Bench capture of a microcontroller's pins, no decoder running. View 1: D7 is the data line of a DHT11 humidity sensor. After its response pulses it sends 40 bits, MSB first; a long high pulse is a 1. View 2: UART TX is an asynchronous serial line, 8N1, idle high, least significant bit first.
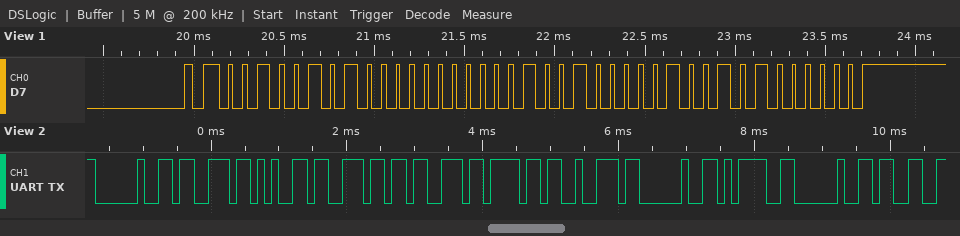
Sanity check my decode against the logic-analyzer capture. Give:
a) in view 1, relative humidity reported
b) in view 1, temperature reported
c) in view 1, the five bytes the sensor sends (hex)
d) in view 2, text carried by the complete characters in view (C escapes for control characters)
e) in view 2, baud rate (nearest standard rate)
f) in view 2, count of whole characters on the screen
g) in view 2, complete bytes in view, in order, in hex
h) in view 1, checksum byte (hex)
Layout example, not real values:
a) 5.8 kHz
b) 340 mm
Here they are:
a) 37 %
b) 18.9 °C
c) 25 00 12 09 40
d) " sensor = 3"
e) 9600 baud
f) 11
g) 20 73 65 6E 73 6F 72 20 3D 20 33
h) 0x40
